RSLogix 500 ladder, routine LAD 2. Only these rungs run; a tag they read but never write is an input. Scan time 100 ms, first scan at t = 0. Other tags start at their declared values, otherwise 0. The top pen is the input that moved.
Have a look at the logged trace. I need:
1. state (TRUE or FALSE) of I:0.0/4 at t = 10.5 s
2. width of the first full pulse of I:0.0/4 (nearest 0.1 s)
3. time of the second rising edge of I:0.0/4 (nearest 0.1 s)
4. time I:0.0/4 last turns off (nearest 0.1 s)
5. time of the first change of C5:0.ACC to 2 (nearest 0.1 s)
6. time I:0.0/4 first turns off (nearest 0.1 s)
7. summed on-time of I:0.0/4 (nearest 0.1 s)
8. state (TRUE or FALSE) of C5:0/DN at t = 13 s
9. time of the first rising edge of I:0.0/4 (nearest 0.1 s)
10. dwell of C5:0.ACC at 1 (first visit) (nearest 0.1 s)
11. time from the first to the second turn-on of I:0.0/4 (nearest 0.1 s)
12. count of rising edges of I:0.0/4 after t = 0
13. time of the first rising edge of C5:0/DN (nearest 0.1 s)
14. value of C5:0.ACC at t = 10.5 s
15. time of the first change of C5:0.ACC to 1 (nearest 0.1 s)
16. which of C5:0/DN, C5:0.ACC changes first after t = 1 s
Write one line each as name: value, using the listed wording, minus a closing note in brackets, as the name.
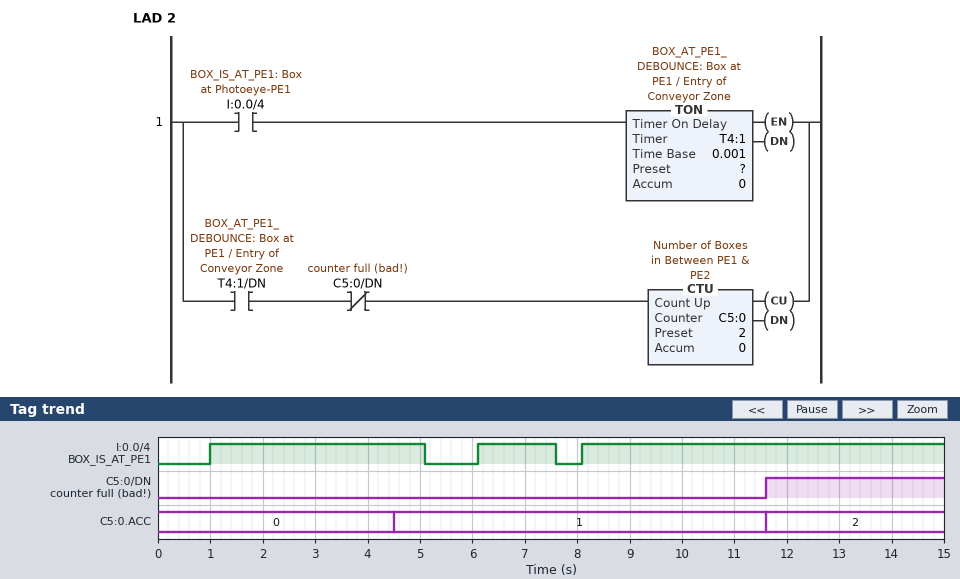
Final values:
state (TRUE or FALSE) of I:0.0/4 at t = 10.5 s: TRUE
width of the first full pulse of I:0.0/4: 4.1 s
time of the second rising edge of I:0.0/4: 6.1 s
time I:0.0/4 last turns off: 7.6 s
time of the first change of C5:0.ACC to 2: 11.6 s
time I:0.0/4 first turns off: 5.1 s
summed on-time of I:0.0/4: 12.5 s
state (TRUE or FALSE) of C5:0/DN at t = 13 s: TRUE
time of the first rising edge of I:0.0/4: 1.0 s
dwell of C5:0.ACC at 1 (first visit): 7.1 s
time from the first to the second turn-on of I:0.0/4: 5.1 s
count of rising edges of I:0.0/4 after t = 0: 3
time of the first rising edge of C5:0/DN: 11.6 s
value of C5:0.ACC at t = 10.5 s: 1
time of the first change of C5:0.ACC to 1: 4.5 s
which of C5:0/DN, C5:0.ACC changes first after t = 1 s: C5:0.ACC
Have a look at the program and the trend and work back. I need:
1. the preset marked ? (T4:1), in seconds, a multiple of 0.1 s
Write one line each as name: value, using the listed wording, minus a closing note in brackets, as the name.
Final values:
the preset marked ? (T4:1), in seconds, a multiple of 0.1 s: 3.5 s
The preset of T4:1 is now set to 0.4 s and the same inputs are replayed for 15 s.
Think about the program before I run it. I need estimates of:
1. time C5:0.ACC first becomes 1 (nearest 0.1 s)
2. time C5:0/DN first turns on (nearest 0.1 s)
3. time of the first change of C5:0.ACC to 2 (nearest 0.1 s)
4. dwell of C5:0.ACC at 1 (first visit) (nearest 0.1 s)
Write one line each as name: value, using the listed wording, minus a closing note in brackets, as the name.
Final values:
time C5:0.ACC first becomes 1: 1.4 s
time C5:0/DN first turns on: 6.5 s
time of the first change of C5:0.ACC to 2: 6.5 s
dwell of C5:0.ACC at 1 (first visit): 5.1 s
